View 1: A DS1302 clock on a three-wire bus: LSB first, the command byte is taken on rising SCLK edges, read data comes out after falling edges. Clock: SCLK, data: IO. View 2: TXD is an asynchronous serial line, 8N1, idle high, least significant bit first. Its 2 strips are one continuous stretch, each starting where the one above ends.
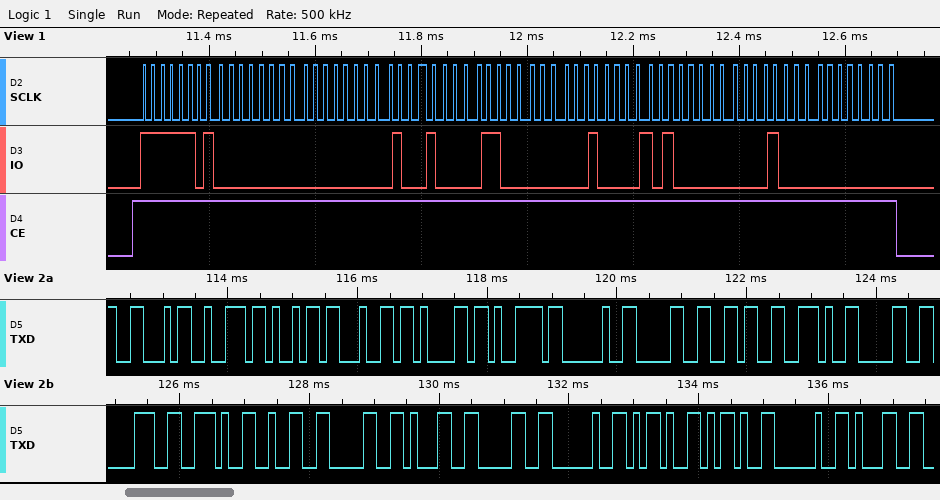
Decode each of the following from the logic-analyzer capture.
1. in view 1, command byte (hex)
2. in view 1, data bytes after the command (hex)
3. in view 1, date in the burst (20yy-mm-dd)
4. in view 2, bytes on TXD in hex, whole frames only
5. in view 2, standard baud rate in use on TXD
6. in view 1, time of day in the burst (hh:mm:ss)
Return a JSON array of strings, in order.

["0xBF", "00 00 12 06 08 05 10 00", "2010-08-06", "46 72 69 64 61 79 20 30 36 2E 30 38 2E 32 30 31 30 20 2D 2D 20 31", "9600 baud", "12:00:00"]
